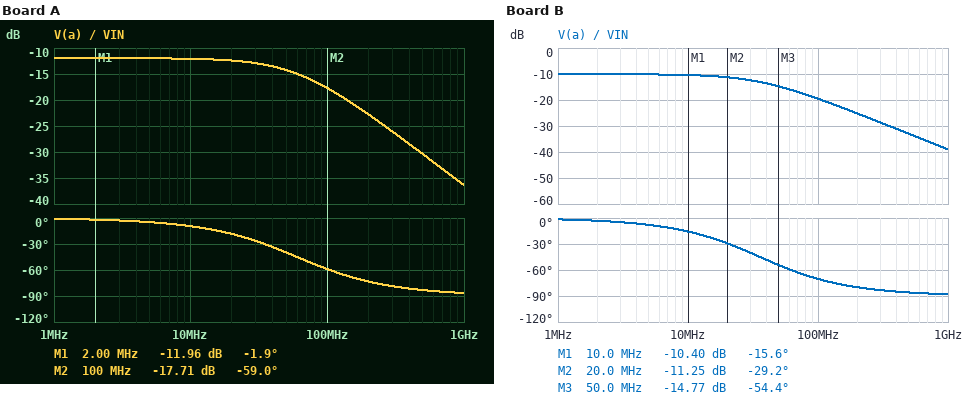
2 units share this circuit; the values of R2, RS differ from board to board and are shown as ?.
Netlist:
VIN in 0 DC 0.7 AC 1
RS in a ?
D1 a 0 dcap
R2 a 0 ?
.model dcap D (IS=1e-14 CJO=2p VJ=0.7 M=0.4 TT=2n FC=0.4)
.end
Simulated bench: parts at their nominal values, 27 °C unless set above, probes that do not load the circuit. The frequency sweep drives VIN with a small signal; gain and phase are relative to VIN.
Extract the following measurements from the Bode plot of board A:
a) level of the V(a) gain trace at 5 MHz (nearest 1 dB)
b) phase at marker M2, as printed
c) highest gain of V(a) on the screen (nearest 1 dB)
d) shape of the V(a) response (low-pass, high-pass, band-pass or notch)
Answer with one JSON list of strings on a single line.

["-12 dB", "-59.0 deg", "-12 dB", "low-pass"]
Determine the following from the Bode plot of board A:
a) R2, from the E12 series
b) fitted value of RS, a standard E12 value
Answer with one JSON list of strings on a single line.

["18 kΩ", "1.5 kΩ"]
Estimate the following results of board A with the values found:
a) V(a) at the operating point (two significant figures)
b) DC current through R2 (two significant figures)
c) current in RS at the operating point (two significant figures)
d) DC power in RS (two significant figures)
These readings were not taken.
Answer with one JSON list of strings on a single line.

["580 mV", "32 µA", "82 µA", "10 µW"]
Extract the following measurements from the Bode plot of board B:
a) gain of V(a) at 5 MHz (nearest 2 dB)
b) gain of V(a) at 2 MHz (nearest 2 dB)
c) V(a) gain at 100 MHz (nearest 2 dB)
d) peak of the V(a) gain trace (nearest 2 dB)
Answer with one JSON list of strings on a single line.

["-10 dB", "-10 dB", "-20 dB", "-10 dB"]
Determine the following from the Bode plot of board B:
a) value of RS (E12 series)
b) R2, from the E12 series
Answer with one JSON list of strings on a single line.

["3.3 kΩ", "18 kΩ"]
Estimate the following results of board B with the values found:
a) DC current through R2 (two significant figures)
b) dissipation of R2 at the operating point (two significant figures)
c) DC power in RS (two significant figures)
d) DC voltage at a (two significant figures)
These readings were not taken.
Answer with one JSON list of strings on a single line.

["30 µA", "17 µW", "7.0 µW", "550 mV"]
